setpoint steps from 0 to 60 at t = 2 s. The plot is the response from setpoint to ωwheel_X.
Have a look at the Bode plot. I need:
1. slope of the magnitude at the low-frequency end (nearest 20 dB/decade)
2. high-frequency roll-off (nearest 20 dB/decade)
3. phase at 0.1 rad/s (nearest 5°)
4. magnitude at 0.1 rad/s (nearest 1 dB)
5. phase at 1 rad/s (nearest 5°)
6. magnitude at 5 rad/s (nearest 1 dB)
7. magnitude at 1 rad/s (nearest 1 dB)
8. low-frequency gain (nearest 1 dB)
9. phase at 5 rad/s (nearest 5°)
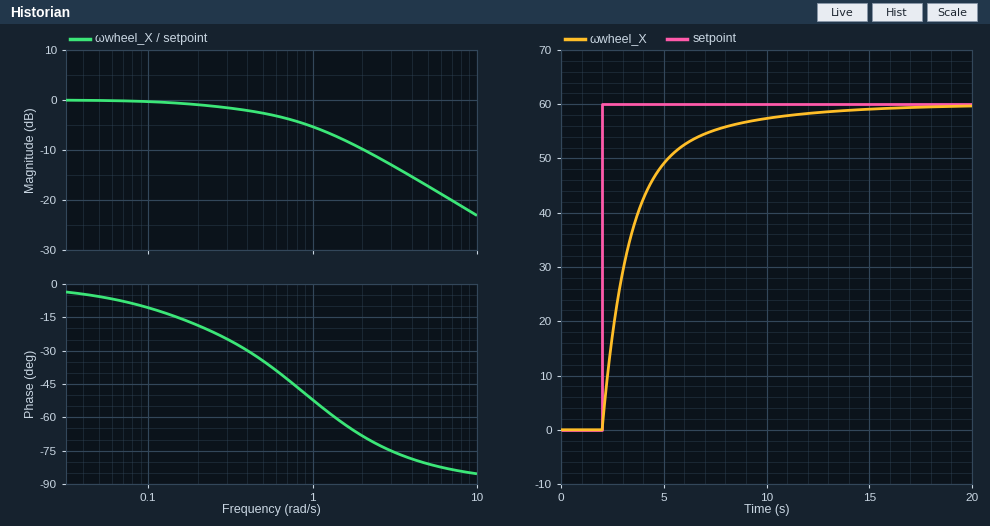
0 dB/decade
-20 dB/decade
-10°
0 dB
-50°
-17 dB
-5 dB
0 dB
-80°
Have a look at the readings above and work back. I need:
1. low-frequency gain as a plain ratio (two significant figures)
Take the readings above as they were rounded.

1.0
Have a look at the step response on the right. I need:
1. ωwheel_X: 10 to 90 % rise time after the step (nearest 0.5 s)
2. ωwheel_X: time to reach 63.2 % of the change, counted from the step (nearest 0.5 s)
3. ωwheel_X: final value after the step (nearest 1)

4.5 s
1.5 s
60
